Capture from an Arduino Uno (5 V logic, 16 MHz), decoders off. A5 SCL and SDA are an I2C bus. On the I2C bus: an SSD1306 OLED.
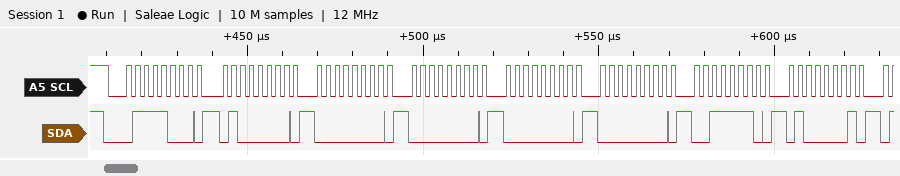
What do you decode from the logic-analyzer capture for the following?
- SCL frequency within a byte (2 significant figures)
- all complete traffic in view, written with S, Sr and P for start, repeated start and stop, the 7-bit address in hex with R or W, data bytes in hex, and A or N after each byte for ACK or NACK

400 kHz
S 3CW A 40 A 00 A 00 A 00 A 00 A 3E A 41 A
